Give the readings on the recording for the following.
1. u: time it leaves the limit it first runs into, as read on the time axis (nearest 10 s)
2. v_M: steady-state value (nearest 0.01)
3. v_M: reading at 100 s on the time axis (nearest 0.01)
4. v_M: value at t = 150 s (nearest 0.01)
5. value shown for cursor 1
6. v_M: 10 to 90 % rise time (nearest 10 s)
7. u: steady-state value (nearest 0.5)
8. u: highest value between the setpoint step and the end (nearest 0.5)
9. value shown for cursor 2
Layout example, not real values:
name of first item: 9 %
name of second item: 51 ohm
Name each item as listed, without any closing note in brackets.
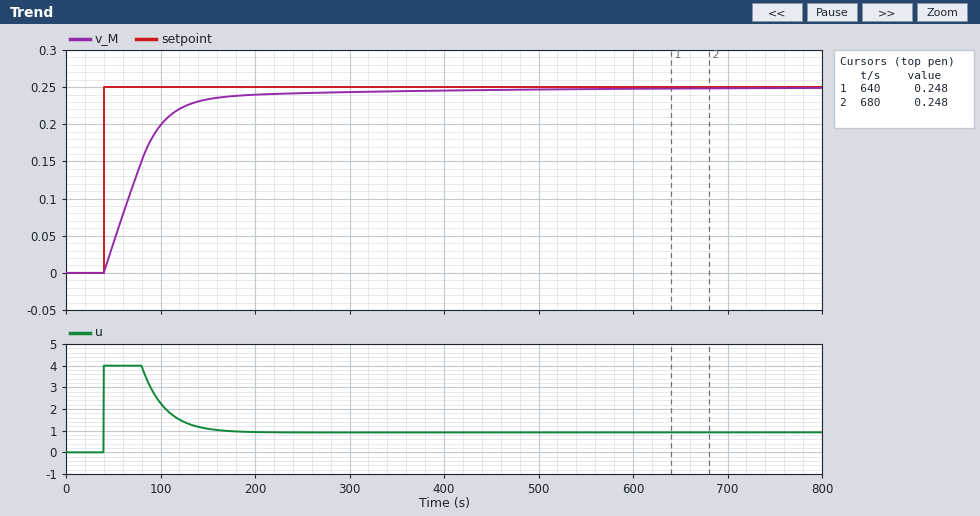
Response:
u: time it leaves the limit it first runs into, as read on the time axis: 80 s
v_M: steady-state value: 0.25
v_M: reading at 100 s on the time axis: 0.20
v_M: value at t = 150 s: 0.23
value shown for cursor 1: 0.248
v_M: 10 to 90 % rise time: 80 s
u: steady-state value: 1.0
u: highest value between the setpoint step and the end: 4.0
value shown for cursor 2: 0.248
